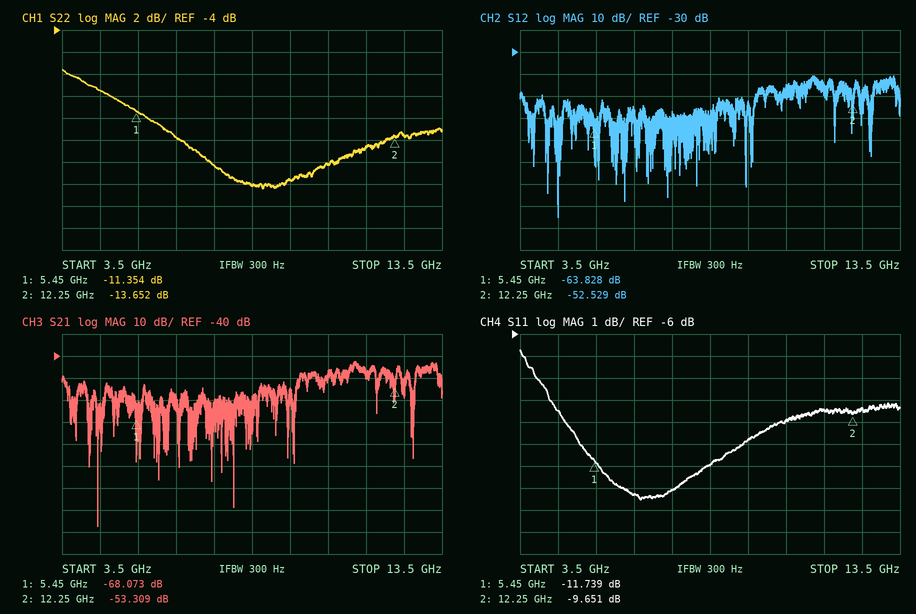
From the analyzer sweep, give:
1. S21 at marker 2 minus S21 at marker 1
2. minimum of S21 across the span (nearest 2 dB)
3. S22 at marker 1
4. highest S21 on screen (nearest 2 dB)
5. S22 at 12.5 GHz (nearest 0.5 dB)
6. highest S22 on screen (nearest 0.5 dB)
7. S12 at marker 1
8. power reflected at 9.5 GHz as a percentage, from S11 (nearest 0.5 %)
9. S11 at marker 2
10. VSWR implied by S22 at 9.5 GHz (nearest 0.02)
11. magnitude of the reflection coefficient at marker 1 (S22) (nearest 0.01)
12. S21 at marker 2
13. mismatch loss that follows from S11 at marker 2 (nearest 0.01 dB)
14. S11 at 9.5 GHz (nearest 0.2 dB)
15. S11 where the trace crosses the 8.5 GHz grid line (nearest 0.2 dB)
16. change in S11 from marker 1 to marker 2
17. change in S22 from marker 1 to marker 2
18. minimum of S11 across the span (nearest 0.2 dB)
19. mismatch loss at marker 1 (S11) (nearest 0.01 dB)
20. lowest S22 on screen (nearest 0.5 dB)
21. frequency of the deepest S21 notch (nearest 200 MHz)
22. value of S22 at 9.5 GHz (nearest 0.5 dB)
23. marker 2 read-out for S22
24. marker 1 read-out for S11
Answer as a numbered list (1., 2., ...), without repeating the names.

1. 14.764 dB
2. -118 dB
3. -11.354 dB
4. -42 dB
5. -13.5 dB
6. -7.5 dB
7. -63.828 dB
8. 8.5 %
9. -9.651 dB
10. 1.30
11. 0.27
12. -53.309 dB
13. 0.50 dB
14. -10.8 dB
15. -12.0 dB
16. 2.088 dB
17. -2.298 dB
18. -13.6 dB
19. 0.30 dB
20. -18.5 dB
21. 4.4 GHz
22. -17.5 dB
23. -13.652 dB
24. -11.739 dB
